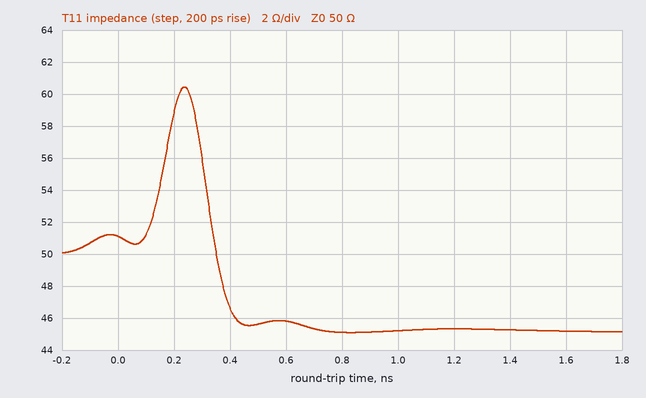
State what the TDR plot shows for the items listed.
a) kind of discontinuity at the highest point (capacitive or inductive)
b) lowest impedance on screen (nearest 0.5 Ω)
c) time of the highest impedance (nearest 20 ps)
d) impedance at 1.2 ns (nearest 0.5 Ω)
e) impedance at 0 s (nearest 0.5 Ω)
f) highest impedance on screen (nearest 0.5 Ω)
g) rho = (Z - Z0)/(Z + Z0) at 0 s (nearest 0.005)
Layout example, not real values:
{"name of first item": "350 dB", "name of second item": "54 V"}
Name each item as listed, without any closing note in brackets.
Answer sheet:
{"kind of discontinuity at the highest point": "inductive", "lowest impedance on screen": "45.0 Ω", "time of the highest impedance": "240 ps", "impedance at 1.2 ns": "45.5 Ω", "impedance at 0 s": "51.0 Ω", "highest impedance on screen": "60.5 Ω", "rho = (Z - Z0)/(Z + Z0) at 0 s": "+0.010"}
